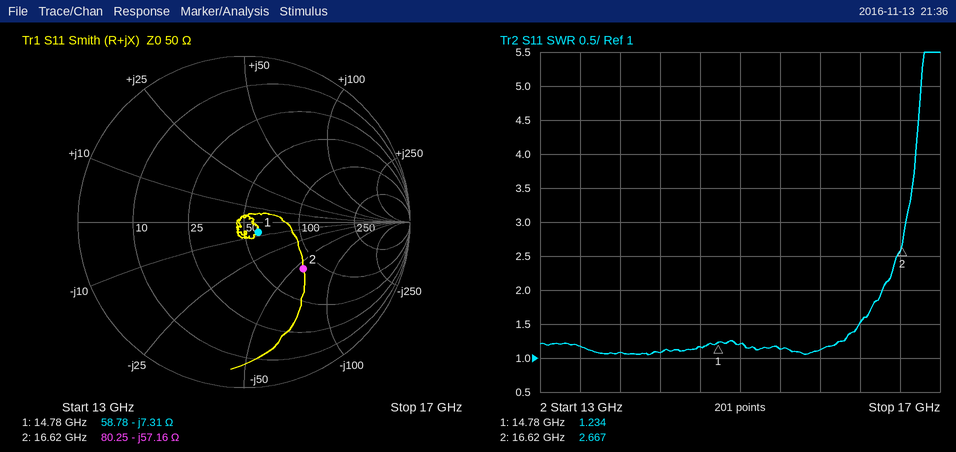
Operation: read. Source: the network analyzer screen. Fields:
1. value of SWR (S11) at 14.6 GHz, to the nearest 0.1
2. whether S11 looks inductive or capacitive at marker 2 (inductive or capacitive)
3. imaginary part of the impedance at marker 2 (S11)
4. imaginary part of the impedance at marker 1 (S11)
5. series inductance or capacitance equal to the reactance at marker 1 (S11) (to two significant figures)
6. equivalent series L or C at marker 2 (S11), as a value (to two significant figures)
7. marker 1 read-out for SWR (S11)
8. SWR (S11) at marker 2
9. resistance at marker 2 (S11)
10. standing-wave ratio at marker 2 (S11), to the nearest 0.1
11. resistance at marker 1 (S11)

1.2
capacitive
-57.16 Ω
-7.31 Ω
1.5 pF
170 fF
1.234
2.667
80.25 Ω
2.7
58.78 Ω
